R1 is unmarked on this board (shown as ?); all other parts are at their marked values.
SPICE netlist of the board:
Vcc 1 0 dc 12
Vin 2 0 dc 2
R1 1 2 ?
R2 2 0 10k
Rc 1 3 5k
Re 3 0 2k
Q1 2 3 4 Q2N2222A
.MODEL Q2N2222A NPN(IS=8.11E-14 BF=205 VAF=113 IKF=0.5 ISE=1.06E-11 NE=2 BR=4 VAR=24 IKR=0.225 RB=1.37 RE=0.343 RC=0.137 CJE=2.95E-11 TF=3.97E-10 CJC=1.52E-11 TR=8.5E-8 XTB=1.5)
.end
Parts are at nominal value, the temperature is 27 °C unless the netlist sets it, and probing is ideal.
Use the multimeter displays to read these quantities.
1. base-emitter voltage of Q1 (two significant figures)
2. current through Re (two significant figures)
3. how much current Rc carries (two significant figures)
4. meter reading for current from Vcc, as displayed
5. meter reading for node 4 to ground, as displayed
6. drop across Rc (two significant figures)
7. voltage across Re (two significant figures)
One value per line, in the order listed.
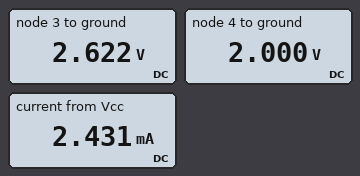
620 mV
1.3 mA
1.9 mA
2.431 mA
2.000 V
9.4 V
2.6 V
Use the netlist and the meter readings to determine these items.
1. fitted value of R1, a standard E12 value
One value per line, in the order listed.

18 kΩ
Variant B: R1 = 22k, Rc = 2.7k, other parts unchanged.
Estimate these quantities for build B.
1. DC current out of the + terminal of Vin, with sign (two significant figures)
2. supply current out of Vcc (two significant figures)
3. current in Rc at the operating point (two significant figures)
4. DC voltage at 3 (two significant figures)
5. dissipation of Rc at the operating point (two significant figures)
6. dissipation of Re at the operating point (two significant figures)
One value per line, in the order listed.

-2.4 mA
3.9 mA
3.5 mA
2.7 V
32 mW
3.5 mW
